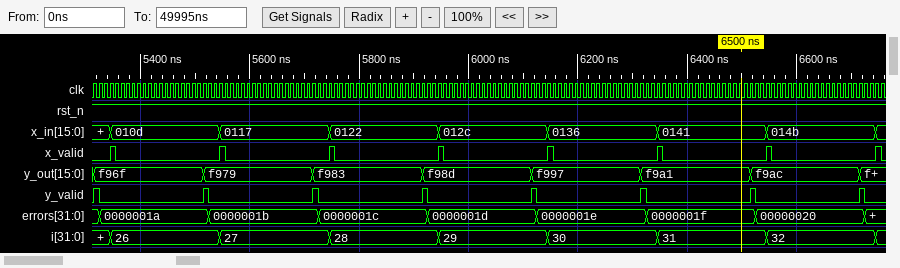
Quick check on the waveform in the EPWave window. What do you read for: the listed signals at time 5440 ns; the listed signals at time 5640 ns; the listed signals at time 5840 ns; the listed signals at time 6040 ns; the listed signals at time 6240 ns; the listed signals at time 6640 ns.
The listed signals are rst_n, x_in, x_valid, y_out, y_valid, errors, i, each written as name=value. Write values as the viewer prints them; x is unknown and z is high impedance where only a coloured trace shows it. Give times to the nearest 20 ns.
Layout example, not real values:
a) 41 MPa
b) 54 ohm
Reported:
a) rst_n=1, x_in=010d, x_valid=0, y_out=f96f, y_valid=0, errors=0000001a, i=26
b) rst_n=1, x_in=0117, x_valid=0, y_out=f979, y_valid=0, errors=0000001b, i=27
c) rst_n=1, x_in=0122, x_valid=0, y_out=f983, y_valid=0, errors=0000001c, i=28
d) rst_n=1, x_in=012c, x_valid=0, y_out=f98d, y_valid=0, errors=0000001d, i=29
e) rst_n=1, x_in=0136, x_valid=0, y_out=f997, y_valid=0, errors=0000001e, i=30
f) rst_n=1, x_in=014b, x_valid=0, y_out=f9ac, y_valid=0, errors=00000020, i=32
